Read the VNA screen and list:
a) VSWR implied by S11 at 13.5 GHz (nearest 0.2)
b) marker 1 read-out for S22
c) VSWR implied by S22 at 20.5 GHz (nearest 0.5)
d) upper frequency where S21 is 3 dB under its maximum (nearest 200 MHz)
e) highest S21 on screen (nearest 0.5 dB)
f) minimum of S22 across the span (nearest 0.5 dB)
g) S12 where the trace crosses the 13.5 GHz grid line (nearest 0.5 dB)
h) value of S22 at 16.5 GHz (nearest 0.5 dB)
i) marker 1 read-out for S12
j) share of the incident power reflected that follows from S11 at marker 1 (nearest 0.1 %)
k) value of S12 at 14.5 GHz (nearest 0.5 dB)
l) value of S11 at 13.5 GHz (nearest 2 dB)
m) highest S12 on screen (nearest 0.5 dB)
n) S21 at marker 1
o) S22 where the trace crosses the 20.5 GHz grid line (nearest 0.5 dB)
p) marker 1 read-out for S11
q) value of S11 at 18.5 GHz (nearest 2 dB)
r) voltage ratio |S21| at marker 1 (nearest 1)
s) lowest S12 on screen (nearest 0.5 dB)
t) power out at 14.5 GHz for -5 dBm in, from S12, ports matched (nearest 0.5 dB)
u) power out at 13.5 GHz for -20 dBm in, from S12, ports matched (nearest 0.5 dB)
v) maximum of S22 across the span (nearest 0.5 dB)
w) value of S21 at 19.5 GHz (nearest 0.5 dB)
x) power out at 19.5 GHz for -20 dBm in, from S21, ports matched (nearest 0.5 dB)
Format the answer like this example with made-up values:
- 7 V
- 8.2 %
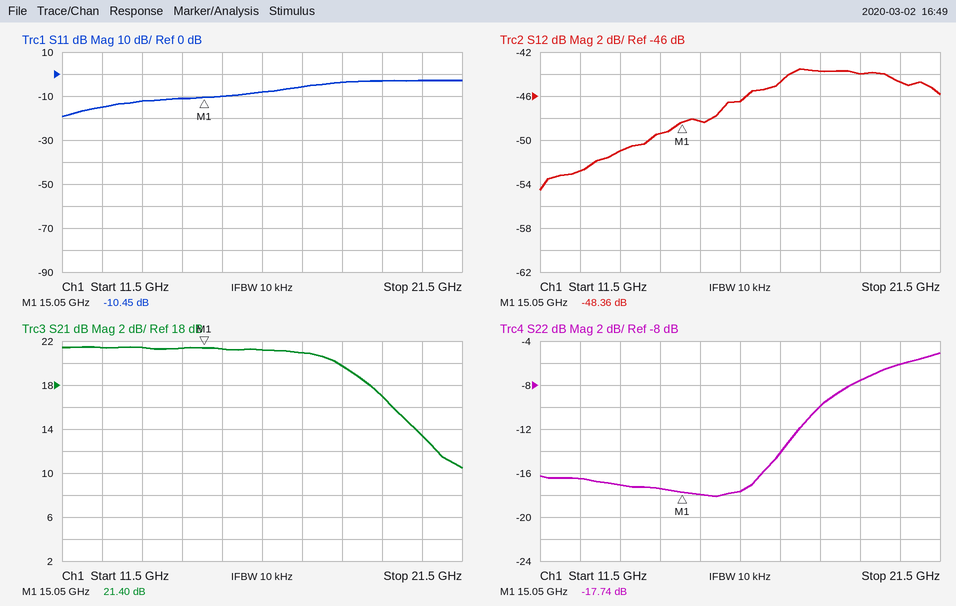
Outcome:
- 1.6
- -17.74 dB
- 3.0
- 19.0 GHz
- 21.5 dB
- -18.0 dB
- -51.0 dB
- -17.5 dB
- -48.36 dB
- 9.0 %
- -49.5 dB
- -12 dB
- -43.5 dB
- 21.40 dB
- -6.0 dB
- -10.45 dB
- -4 dB
- 12
- -54.5 dB
- -54.5 dBm
- -71.0 dBm
- -5.0 dB
- 17.0 dB
- -3.0 dBm
